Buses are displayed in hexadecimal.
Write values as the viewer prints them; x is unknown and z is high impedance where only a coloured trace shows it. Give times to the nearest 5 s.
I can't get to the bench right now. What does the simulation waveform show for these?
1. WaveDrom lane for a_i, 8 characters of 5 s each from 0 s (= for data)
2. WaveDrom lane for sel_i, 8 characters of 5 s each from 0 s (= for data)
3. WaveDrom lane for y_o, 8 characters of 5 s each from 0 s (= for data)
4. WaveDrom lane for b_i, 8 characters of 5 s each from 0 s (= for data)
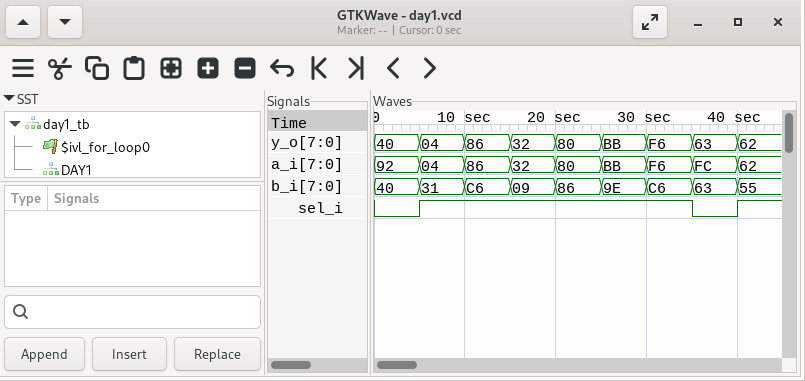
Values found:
{name: 'a_i', wave: '========', data: '92 04 86 32 80 BB F6 FC'}
{name: 'sel_i', wave: '01.....0'}
{name: 'y_o', wave: '========', data: '40 04 86 32 80 BB F6 63'}
{name: 'b_i', wave: '========', data: '40 31 C6 09 86 9E C6 63'}
